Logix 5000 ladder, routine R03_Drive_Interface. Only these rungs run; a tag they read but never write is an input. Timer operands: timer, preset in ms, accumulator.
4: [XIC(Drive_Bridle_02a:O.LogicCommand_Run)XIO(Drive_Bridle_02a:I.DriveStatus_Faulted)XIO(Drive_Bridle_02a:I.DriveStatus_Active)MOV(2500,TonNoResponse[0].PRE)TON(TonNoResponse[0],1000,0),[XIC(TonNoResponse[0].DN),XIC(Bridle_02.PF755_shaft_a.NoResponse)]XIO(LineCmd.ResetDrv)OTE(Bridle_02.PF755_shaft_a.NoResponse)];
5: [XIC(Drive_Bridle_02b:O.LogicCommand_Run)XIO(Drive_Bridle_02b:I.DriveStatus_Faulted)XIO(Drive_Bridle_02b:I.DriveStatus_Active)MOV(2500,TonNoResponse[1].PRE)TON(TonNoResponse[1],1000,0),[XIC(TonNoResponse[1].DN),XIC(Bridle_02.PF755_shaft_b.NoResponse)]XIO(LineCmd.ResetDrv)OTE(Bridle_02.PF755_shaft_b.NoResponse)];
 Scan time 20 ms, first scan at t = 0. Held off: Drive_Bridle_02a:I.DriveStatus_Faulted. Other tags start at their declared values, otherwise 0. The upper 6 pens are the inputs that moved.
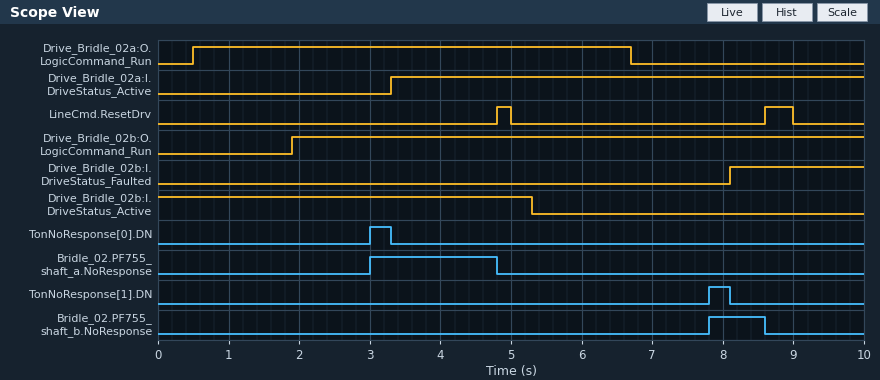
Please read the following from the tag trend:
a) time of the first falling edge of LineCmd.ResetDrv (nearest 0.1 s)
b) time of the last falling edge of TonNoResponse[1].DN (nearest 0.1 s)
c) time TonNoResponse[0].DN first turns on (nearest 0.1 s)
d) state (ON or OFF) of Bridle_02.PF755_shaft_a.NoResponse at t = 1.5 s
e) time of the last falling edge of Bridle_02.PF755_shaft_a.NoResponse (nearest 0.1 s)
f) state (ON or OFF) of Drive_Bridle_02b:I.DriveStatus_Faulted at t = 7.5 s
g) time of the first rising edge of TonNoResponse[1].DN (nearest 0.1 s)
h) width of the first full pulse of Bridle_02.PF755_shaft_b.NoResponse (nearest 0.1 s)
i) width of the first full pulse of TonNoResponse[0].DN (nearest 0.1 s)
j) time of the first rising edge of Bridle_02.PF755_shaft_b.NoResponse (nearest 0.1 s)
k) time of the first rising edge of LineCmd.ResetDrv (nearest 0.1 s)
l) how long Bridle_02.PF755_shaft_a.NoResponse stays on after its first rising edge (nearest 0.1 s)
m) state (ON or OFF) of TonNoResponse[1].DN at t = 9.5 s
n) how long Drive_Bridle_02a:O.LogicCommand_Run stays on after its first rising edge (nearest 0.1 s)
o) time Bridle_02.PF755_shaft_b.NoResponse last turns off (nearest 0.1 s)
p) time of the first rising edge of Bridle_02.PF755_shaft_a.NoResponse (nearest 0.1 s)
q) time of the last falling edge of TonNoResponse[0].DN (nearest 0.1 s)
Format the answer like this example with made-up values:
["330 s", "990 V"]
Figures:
["5.0 s", "8.1 s", "3.0 s", "OFF", "4.8 s", "OFF", "7.8 s", "0.8 s", "0.3 s", "7.8 s", "4.8 s", "1.8 s", "OFF", "6.2 s", "8.6 s", "3.0 s", "3.3 s"]
